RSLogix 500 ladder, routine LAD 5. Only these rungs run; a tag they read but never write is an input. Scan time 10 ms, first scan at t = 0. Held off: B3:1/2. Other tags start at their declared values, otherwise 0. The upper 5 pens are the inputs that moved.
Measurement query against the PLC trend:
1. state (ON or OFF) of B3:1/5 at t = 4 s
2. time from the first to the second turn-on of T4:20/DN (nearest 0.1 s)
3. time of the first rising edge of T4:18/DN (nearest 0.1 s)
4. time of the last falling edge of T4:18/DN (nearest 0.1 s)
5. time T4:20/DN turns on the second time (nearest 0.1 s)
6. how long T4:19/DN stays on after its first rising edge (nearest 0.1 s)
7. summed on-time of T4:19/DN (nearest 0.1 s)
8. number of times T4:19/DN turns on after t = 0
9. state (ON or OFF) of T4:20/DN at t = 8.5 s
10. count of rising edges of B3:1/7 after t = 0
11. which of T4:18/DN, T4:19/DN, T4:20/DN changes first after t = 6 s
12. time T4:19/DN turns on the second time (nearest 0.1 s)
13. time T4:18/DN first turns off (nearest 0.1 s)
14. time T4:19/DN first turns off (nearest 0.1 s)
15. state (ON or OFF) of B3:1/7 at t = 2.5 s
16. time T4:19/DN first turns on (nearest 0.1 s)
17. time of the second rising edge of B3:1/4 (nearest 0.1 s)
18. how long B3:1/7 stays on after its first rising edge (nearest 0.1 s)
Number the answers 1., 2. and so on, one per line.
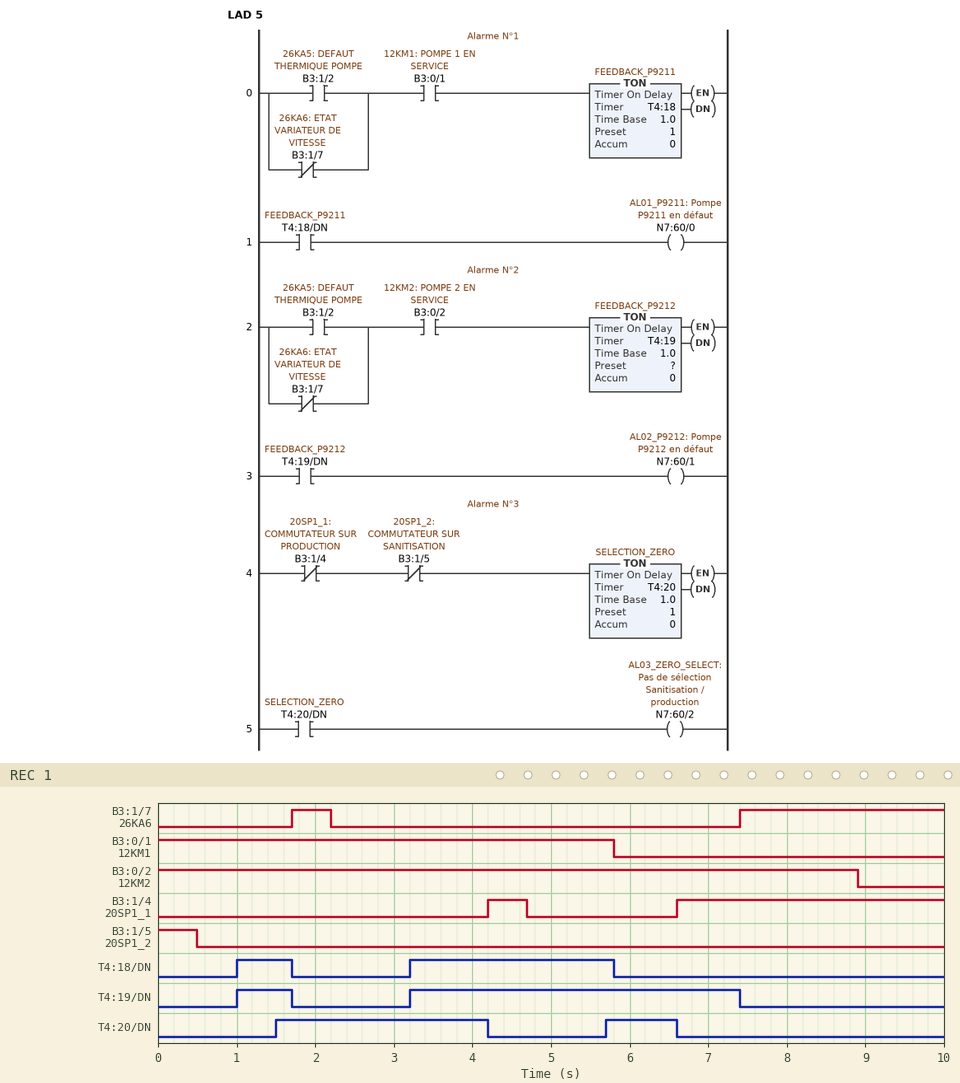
1. OFF
2. 4.2 s
3. 1.0 s
4. 5.8 s
5. 5.7 s
6. 0.7 s
7. 4.9 s
8. 2
9. OFF
10. 2
11. T4:20/DN
12. 3.2 s
13. 1.7 s
14. 1.7 s
15. OFF
16. 1.0 s
17. 6.6 s
18. 0.5 s
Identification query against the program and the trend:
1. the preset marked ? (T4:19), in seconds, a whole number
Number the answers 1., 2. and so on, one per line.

1. 1 s
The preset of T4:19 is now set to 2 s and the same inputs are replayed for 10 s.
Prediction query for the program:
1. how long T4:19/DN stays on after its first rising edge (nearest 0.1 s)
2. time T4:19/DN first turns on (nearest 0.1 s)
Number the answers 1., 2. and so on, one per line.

1. 3.2 s
2. 4.2 s
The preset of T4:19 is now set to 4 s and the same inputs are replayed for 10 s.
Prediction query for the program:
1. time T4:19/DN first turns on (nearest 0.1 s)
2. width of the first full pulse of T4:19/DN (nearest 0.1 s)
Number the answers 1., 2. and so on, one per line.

1. 6.2 s
2. 1.2 s
